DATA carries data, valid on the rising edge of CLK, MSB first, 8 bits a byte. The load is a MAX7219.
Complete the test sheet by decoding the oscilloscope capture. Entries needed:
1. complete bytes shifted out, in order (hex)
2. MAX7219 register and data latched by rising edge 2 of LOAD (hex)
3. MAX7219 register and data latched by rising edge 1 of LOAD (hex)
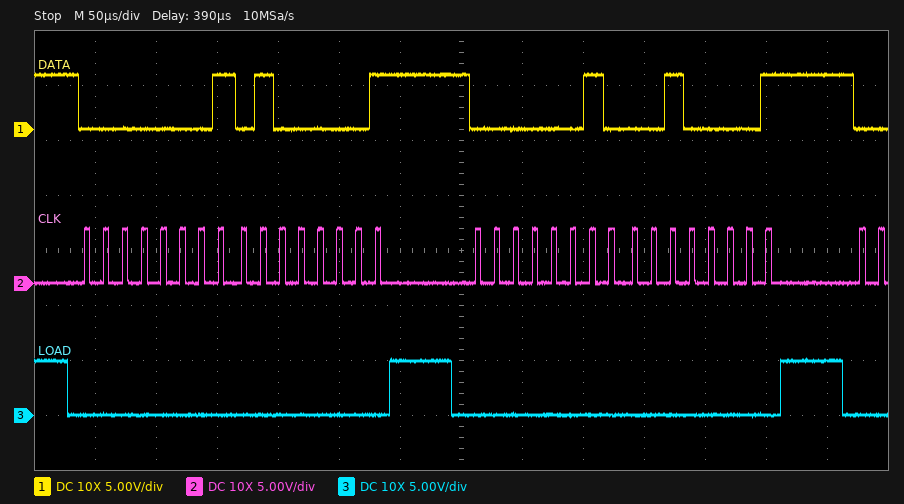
01 41 02 21
register 0x2, data 0x21
register 0x1, data 0x41
